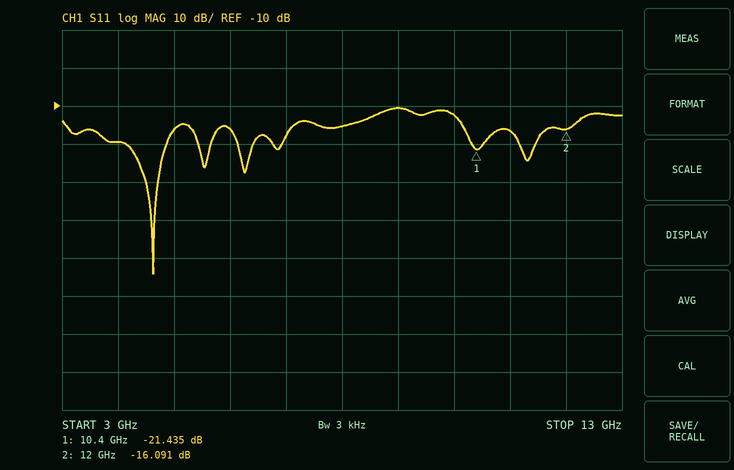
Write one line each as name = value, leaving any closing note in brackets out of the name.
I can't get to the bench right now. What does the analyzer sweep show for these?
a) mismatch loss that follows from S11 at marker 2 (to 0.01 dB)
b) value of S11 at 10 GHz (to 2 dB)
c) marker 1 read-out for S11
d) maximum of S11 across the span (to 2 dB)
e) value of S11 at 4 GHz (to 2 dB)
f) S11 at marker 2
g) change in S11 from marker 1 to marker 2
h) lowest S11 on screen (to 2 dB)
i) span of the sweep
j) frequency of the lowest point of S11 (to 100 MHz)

mismatch loss that follows from S11 at marker 2 = 0.11 dB
value of S11 at 10 GHz = -12 dB
marker 1 read-out for S11 = -21.435 dB
maximum of S11 across the span = -10 dB
value of S11 at 4 GHz = -20 dB
S11 at marker 2 = -16.091 dB
change in S11 from marker 1 to marker 2 = 5.344 dB
lowest S11 on screen = -54 dB
span of the sweep = 10 GHz
frequency of the lowest point of S11 = 4.6 GHz
